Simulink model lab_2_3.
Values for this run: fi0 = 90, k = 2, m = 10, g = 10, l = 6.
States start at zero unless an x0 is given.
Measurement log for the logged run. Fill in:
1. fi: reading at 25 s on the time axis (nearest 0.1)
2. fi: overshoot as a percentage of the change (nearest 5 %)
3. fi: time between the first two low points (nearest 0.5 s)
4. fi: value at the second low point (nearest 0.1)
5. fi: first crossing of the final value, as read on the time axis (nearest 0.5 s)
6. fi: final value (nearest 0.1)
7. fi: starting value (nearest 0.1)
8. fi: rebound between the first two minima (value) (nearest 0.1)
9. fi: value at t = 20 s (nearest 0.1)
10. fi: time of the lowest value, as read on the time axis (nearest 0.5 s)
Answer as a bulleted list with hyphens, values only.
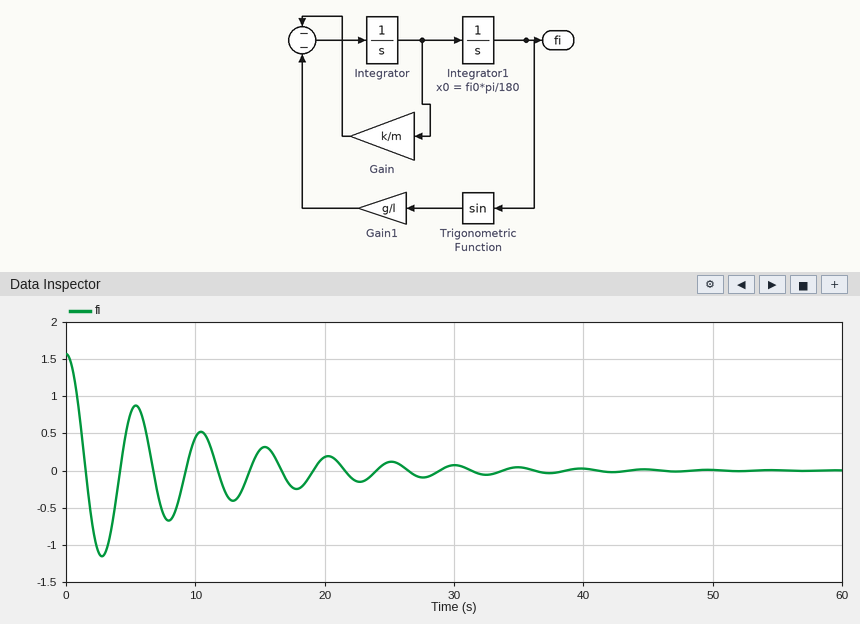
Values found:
- 0.1
- 75 %
- 5.0 s
- -0.7
- 1.5 s
- 0.0
- 1.6
- 0.9
- 0.2
- 3.0 s
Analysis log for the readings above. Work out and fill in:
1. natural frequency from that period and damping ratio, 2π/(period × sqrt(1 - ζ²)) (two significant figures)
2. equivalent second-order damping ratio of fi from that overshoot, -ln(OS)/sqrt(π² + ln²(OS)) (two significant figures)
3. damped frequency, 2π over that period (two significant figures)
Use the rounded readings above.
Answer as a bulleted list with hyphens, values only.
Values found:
- 1.3 rad/s
- 0.091
- 1.3 rad/s
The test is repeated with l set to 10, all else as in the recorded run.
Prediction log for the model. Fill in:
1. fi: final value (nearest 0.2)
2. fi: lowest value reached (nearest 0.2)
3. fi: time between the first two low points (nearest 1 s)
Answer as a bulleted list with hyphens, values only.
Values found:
- 0.0
- -1.0
- 7 s
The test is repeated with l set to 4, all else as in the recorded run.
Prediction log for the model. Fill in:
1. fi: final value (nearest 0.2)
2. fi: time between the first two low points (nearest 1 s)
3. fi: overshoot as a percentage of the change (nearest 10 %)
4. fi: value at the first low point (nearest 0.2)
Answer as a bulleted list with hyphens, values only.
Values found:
- 0.0
- 4 s
- 80 %
- -1.2
